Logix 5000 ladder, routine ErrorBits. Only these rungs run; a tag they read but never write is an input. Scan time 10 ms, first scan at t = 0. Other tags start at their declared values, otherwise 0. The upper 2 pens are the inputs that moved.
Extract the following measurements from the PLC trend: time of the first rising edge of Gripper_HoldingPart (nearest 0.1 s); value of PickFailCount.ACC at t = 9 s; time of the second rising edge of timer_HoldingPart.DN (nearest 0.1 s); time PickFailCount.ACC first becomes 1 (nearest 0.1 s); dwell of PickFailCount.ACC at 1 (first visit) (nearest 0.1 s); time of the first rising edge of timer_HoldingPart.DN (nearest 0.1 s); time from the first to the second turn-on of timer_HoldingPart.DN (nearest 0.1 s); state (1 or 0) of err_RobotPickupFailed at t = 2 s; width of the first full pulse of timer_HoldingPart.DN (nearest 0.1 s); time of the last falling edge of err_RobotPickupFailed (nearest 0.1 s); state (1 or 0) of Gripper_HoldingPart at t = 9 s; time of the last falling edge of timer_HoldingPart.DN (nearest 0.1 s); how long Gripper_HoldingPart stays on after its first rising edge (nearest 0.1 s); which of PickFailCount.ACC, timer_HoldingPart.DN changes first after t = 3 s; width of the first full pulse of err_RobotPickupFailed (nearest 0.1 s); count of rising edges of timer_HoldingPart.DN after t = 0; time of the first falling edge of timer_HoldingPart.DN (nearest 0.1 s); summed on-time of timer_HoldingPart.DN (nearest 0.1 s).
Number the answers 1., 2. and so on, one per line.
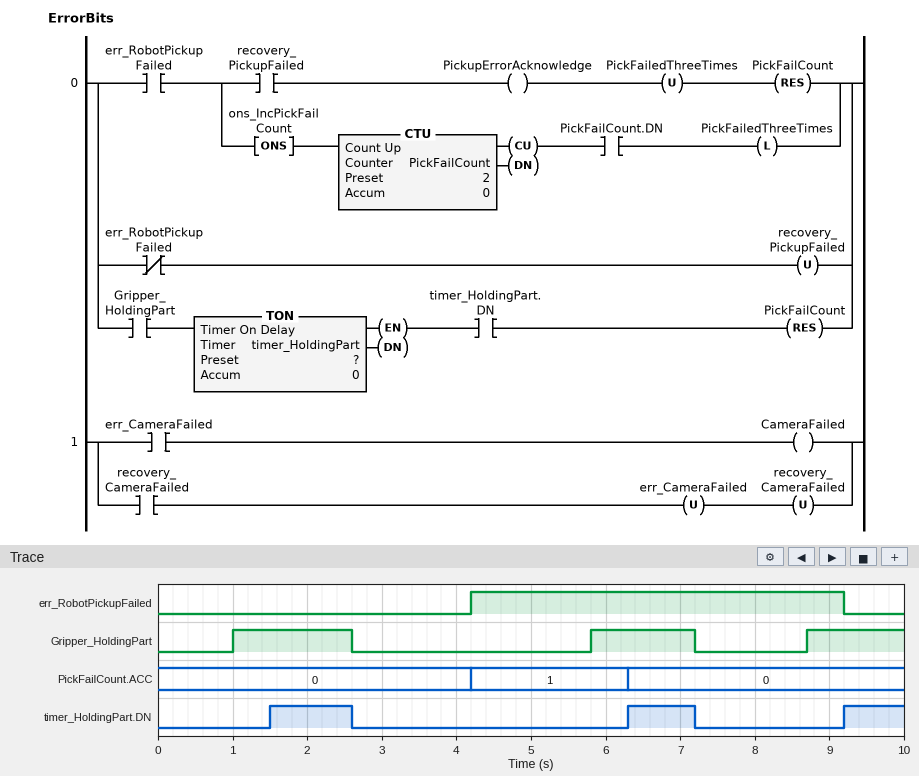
1. 1.0 s
2. 0
3. 6.3 s
4. 4.2 s
5. 2.1 s
6. 1.5 s
7. 4.8 s
8. 0
9. 1.1 s
10. 9.2 s
11. 1
12. 7.2 s
13. 1.6 s
14. PickFailCount.ACC
15. 5.0 s
16. 3
17. 2.6 s
18. 2.8 s
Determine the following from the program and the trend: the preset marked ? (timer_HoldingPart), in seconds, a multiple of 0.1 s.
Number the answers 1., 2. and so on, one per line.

1. 0.5 s
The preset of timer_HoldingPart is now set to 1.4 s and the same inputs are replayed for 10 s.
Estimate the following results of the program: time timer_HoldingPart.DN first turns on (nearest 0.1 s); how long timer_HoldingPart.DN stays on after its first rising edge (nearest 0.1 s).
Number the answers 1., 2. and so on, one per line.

1. 2.4 s
2. 0.2 s
